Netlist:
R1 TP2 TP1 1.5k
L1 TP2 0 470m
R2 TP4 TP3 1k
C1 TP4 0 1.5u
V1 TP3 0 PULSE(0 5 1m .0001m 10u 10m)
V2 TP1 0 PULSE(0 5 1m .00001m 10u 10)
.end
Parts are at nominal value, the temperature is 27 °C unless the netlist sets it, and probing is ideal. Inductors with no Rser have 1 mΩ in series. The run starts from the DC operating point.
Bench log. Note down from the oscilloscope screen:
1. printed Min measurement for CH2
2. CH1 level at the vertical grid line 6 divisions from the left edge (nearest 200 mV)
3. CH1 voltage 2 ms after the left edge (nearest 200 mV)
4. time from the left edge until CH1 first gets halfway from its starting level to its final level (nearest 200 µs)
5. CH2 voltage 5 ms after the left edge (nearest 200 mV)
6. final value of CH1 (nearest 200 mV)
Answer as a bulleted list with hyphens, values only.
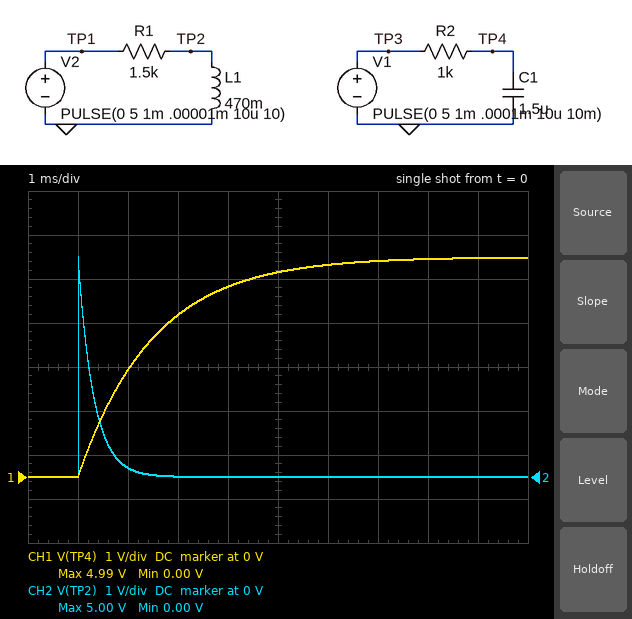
- 0.00 V
- 4.8 V
- 2.4 V
- 2.0 ms
- 0 V
- 5.0 V
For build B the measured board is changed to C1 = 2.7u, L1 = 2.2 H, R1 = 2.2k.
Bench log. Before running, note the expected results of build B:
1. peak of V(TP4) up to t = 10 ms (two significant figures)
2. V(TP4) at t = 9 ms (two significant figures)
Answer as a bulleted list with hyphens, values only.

- 4.8 V
- 4.7 V
